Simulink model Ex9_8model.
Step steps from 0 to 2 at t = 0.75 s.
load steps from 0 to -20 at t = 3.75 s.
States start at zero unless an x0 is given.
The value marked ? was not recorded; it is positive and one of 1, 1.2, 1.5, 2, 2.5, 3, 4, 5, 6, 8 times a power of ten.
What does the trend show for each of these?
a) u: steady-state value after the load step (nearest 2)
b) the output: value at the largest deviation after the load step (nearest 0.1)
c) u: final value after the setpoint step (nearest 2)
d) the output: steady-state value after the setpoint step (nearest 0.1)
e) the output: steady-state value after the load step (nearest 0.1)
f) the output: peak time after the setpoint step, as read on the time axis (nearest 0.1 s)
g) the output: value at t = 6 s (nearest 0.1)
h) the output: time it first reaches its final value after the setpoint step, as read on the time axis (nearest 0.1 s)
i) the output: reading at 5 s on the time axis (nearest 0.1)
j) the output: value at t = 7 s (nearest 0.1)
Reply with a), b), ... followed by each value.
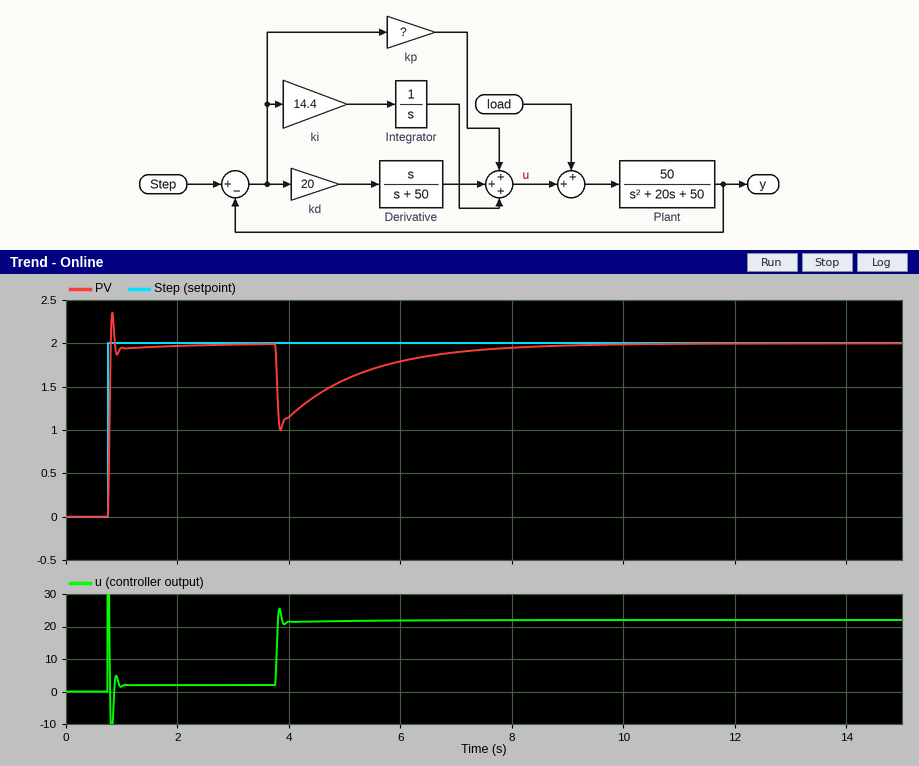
a) 22
b) 1.0
c) 2
d) 2.0
e) 2.0
f) 0.8 s
g) 1.8
h) 0.8 s
i) 1.6
j) 1.9
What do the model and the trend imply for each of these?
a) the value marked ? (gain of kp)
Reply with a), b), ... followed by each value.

a) 20
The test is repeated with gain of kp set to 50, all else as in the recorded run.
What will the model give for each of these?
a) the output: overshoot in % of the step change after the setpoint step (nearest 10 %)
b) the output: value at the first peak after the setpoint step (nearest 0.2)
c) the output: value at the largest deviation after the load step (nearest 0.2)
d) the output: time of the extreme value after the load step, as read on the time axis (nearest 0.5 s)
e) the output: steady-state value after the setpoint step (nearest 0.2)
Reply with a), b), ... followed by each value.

a) 40 %
b) 2.8
c) 1.4
d) 4.0 s
e) 2.0
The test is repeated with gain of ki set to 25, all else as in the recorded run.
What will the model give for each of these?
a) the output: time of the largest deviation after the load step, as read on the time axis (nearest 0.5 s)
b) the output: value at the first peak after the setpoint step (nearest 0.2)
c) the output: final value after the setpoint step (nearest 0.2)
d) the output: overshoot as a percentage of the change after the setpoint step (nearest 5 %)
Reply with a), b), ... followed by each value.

a) 4.0 s
b) 2.4
c) 2.0
d) 20 %
